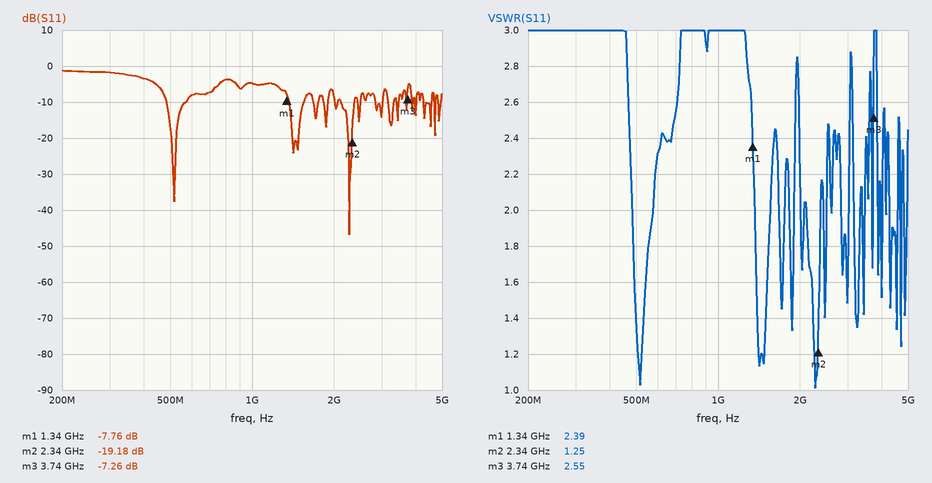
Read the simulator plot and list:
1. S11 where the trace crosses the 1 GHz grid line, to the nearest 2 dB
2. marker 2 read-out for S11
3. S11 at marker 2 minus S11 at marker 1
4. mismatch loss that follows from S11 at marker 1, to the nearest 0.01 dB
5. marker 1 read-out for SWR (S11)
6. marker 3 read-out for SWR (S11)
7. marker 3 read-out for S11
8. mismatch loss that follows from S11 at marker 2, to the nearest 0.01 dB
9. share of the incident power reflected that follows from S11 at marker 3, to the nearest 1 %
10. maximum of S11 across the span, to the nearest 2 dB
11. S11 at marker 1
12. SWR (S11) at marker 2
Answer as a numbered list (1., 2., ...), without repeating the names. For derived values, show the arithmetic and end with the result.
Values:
1. -4 dB
2. -19.18 dB
3. -19.18 − (-7.76) = -11.42 dB
4. −10 log10(1 − 10^(-7.76/10)) ≈ 0.80 dB
5. 2.39
6. 2.55
7. -7.26 dB
8. −10 log10(1 − 10^(-19.18/10)) ≈ 0.05 dB
9. 10^(-7.26/10) ≈ 19 %
10. -2 dB
11. -7.76 dB
12. 1.25
